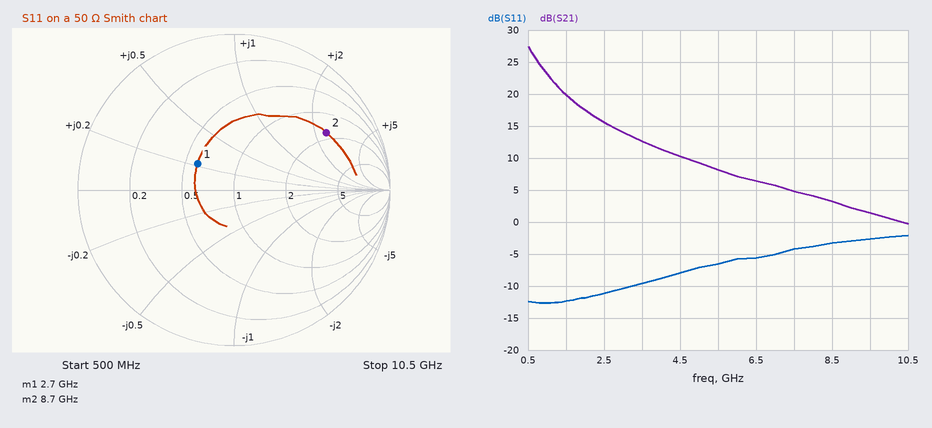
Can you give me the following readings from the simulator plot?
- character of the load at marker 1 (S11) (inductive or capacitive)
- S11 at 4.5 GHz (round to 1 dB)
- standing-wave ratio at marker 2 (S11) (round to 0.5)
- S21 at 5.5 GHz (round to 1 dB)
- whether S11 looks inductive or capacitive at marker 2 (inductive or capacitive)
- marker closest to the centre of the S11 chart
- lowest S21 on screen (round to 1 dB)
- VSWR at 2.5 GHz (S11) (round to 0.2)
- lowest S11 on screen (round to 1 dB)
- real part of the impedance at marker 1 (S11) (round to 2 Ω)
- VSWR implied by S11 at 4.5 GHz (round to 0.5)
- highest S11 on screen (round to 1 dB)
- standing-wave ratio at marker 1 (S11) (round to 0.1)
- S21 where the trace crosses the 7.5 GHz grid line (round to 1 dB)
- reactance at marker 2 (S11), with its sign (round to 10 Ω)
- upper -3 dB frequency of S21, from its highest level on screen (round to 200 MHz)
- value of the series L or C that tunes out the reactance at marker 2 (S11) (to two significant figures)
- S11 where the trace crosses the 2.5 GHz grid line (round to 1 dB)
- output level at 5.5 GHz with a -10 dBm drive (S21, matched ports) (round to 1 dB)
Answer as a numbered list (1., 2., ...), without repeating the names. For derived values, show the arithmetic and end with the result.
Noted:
1. inductive
2. -8 dB
3. 5.5
4. 8 dB
5. inductive
6. marker 1
7. 0 dB
8. |Γ| = 10^(-11/20) = 0.2818; VSWR = (1 + 0.2818)/(1 − 0.2818) ≈ 1.8
9. -13 dB
10. 30 Ω
11. |Γ| = 10^(-8/20) = 0.3981; VSWR = (1 + 0.3981)/(1 − 0.3981) ≈ 2.32, so 2.5 to the nearest 0.5
12. -2 dB
13. 1.8
14. 5 dB
15. +120 Ω
16. 800 MHz
17. C = 1/(2π × 8.7 GHz × 120 Ω) ≈ 152 fF, so 150 fF to two significant figures
18. -11 dB
19. -10 dBm + (8 dB) = -2 dBm
